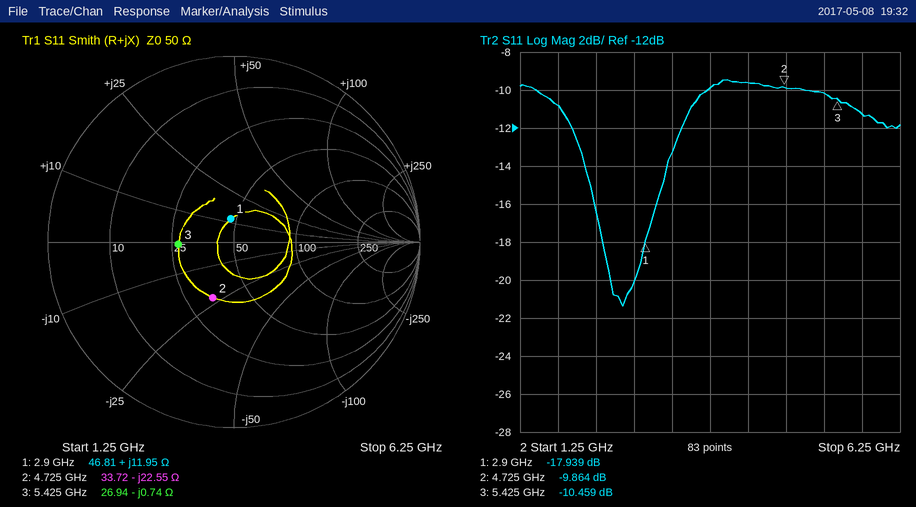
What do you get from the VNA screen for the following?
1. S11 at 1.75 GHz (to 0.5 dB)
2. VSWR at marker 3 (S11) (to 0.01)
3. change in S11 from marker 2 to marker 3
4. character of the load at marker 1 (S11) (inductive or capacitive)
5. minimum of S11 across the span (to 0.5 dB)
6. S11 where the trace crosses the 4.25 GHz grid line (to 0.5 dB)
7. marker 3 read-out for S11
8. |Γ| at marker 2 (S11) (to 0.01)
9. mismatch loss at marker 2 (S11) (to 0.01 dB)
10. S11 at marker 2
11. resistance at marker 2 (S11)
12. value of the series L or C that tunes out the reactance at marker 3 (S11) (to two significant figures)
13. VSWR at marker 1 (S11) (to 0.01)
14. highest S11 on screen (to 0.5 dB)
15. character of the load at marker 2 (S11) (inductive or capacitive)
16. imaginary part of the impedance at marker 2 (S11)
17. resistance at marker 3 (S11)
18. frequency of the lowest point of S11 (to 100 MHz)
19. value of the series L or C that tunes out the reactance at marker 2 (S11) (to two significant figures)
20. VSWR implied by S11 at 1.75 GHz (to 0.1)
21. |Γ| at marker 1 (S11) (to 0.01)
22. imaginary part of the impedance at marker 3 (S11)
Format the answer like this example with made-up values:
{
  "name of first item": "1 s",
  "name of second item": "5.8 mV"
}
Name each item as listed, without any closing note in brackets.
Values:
{
  "S11 at 1.75 GHz": "-11.0 dB",
  "VSWR at marker 3 (S11)": "1.86",
  "change in S11 from marker 2 to marker 3": "-0.595 dB",
  "character of the load at marker 1 (S11)": "inductive",
  "minimum of S11 across the span": "-21.5 dB",
  "S11 where the trace crosses the 4.25 GHz grid line": "-9.5 dB",
  "marker 3 read-out for S11": "-10.459 dB",
  "|Γ| at marker 2 (S11)": "0.32",
  "mismatch loss at marker 2 (S11)": "0.47 dB",
  "S11 at marker 2": "-9.864 dB",
  "resistance at marker 2": "33.72 Ω",
  "value of the series L or C that tunes out the reactance at marker 3 (S11)": "22 pH",
  "VSWR at marker 1 (S11)": "1.29",
  "highest S11 on screen": "-9.5 dB",
  "character of the load at marker 2 (S11)": "capacitive",
  "imaginary part of the impedance at marker 2": "-22.55 Ω",
  "resistance at marker 3": "26.94 Ω",
  "frequency of the lowest point of S11": "2.6 GHz",
  "value of the series L or C that tunes out the reactance at marker 2 (S11)": "760 pH",
  "VSWR implied by S11 at 1.75 GHz": "1.8",
  "|Γ| at marker 1 (S11)": "0.13",
  "imaginary part of the impedance at marker 3": "-0.74 Ω"
}
